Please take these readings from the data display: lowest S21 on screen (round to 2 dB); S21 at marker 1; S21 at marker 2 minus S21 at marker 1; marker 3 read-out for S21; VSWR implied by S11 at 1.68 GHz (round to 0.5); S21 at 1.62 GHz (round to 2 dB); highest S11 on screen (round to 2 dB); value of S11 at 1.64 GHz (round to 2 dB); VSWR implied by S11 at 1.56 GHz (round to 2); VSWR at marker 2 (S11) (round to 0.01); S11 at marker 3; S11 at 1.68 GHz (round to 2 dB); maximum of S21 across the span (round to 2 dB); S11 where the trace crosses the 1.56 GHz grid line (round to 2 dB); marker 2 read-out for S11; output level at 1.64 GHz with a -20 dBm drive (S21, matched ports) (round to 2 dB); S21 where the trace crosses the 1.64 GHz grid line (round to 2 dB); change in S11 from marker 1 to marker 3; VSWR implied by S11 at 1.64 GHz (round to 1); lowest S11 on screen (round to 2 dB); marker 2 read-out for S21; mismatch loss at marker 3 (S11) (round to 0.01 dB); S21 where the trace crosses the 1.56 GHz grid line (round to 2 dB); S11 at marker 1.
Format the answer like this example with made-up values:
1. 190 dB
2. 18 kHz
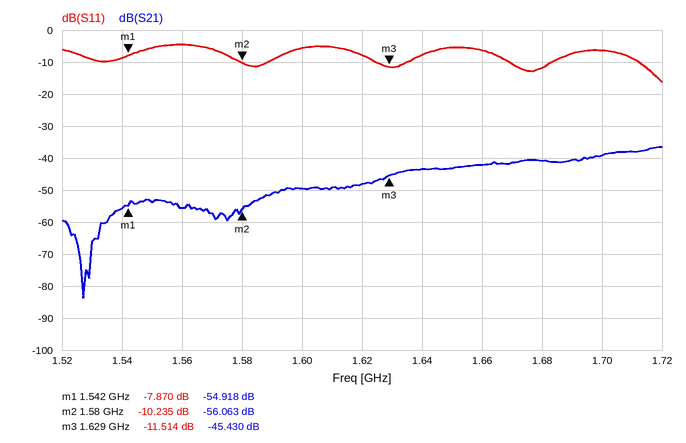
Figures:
1. -84 dB
2. -54.918 dB
3. -1.145 dB
4. -45.430 dB
5. 1.5
6. -48 dB
7. -4 dB
8. -8 dB
9. 4
10. 1.89
11. -11.514 dB
12. -12 dB
13. -36 dB
14. -4 dB
15. -10.235 dB
16. -64 dBm
17. -44 dB
18. -3.644 dB
19. 2
20. -16 dB
21. -56.063 dB
22. 0.32 dB
23. -56 dB
24. -7.870 dB
